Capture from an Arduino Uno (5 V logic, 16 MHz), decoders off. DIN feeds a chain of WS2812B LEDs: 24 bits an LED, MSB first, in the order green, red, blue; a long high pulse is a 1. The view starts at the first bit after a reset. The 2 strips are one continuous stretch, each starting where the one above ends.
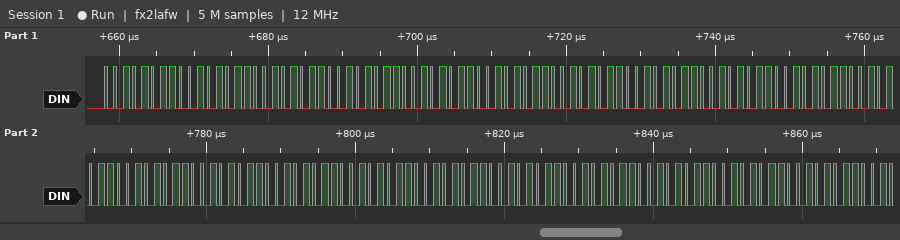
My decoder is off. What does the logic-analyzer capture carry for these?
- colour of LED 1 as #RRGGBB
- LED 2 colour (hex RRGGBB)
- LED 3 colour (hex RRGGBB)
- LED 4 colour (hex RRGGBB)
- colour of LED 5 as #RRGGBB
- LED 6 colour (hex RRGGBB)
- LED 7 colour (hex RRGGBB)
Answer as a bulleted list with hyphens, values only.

- #2B2B2B
- #2B2B2B
- #2B2B2B
- #2B2B2B
- #2B2B2B
- #2B2B2B
- #2B2B2B
